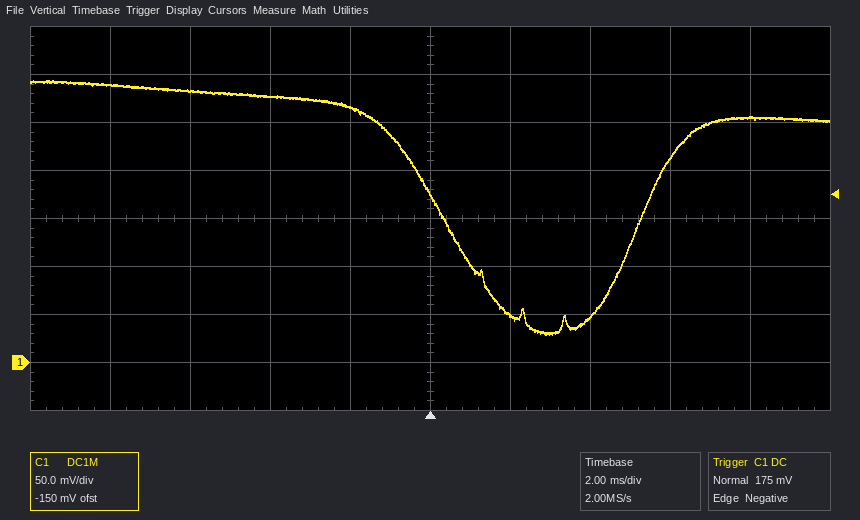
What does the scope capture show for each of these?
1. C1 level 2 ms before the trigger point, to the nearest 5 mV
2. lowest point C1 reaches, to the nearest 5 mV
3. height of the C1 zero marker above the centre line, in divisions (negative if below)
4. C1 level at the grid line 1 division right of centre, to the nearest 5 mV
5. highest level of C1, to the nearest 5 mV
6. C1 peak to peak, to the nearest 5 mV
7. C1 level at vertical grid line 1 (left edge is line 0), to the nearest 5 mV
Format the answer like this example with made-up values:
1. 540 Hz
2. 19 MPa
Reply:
1. 265 mV
2. 30 mV
3. -3.0 div
4. 50 mV
5. 295 mV
6. 265 mV
7. 290 mV
